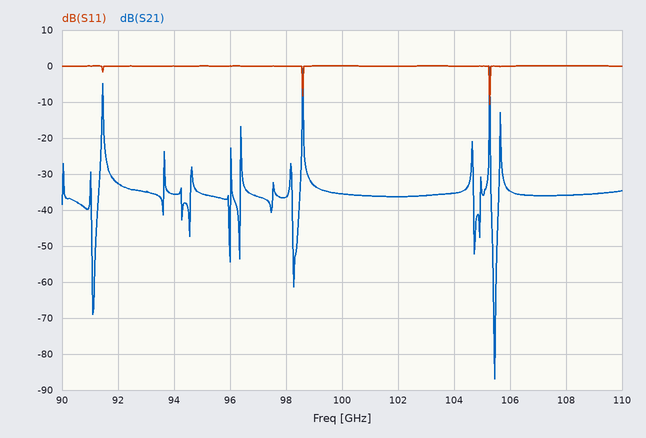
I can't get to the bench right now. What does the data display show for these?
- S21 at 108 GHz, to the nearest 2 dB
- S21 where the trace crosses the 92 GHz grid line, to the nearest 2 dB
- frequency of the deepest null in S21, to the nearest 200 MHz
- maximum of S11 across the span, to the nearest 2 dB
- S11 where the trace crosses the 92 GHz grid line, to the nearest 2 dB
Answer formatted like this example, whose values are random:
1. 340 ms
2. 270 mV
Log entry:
1. -36 dB
2. -32 dB
3. 105.4 GHz
4. 0 dB
5. 0 dB
